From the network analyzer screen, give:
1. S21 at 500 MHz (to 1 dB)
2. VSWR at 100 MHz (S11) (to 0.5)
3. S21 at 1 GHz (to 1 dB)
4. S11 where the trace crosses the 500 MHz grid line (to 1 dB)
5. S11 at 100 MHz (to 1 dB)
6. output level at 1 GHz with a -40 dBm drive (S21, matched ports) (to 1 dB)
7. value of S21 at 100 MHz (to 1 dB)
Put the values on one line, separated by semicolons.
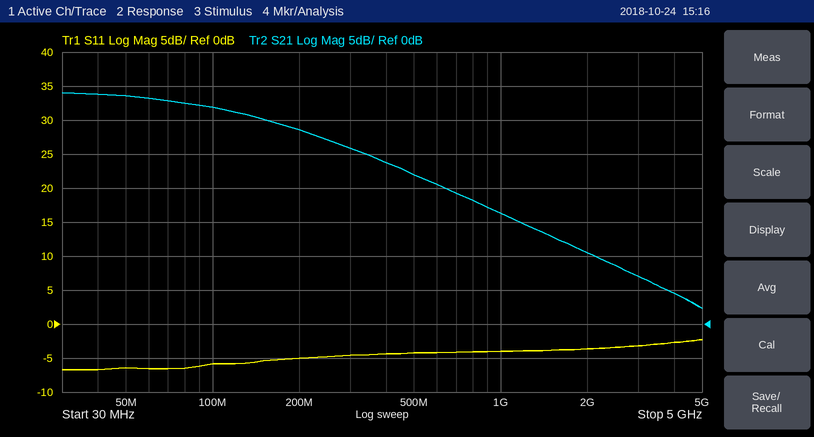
22 dB; 3.0; 16 dB; -4 dB; -6 dB; -24 dBm; 32 dB
